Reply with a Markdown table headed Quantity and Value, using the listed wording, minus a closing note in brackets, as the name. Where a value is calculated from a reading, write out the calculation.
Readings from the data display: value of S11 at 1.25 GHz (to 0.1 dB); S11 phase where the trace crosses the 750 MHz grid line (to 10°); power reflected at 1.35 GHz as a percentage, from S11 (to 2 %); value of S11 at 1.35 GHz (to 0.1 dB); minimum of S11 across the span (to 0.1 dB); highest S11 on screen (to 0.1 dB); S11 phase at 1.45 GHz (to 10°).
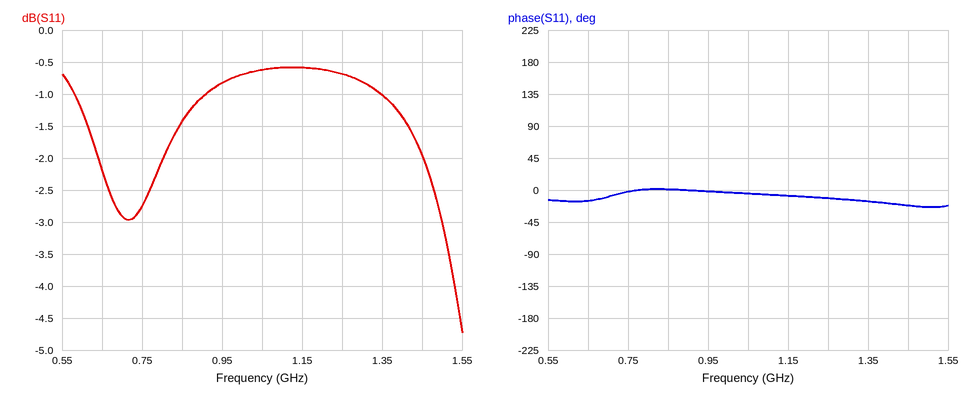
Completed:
| Quantity | Value |
|---|---|
| value of S11 at 1.25 GHz | -0.7 dB |
| S11 phase where the trace crosses the 750 MHz grid line | 0° |
| power reflected at 1.35 GHz as a percentage, from S11 | 10^(-1/10) ≈ 79.4 %, so 80 % to the nearest 2 % |
| value of S11 at 1.35 GHz | -1.0 dB |
| minimum of S11 across the span | -4.7 dB |
| highest S11 on screen | -0.6 dB |
| S11 phase at 1.45 GHz | -20° |
